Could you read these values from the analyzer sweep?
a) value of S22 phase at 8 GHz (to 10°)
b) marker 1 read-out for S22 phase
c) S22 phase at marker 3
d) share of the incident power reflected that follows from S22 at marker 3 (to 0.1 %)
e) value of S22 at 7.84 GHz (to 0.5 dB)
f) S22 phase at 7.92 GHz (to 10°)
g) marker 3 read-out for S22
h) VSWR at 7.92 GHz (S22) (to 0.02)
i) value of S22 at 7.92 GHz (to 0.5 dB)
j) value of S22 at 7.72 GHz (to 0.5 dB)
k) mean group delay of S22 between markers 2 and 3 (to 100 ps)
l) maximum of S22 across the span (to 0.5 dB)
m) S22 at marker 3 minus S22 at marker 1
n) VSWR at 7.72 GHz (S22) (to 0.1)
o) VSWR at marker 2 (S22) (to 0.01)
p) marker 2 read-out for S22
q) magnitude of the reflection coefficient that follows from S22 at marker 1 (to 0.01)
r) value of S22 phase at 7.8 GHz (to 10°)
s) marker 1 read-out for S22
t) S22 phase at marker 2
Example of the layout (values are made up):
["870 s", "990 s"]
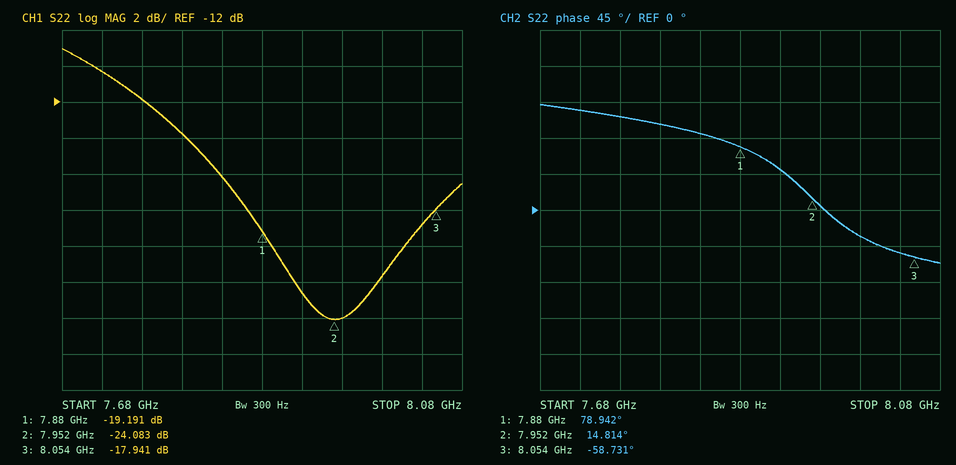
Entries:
["-30°", "78.942°", "-58.731°", "1.6 %", "-16.0 dB", "50°", "-17.941 dB", "1.16", "-22.5 dB", "-10.5 dB", "2.0 ns", "-9.0 dB", "1.250 dB", "1.9", "1.13", "-24.083 dB", "0.11", "110°", "-19.191 dB", "14.814°"]
